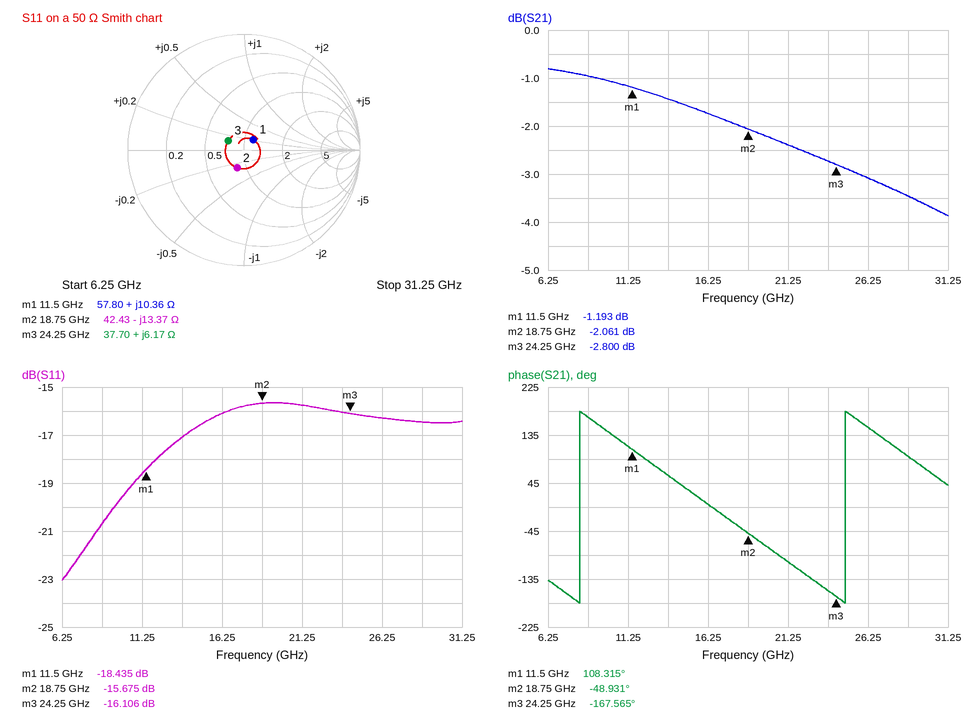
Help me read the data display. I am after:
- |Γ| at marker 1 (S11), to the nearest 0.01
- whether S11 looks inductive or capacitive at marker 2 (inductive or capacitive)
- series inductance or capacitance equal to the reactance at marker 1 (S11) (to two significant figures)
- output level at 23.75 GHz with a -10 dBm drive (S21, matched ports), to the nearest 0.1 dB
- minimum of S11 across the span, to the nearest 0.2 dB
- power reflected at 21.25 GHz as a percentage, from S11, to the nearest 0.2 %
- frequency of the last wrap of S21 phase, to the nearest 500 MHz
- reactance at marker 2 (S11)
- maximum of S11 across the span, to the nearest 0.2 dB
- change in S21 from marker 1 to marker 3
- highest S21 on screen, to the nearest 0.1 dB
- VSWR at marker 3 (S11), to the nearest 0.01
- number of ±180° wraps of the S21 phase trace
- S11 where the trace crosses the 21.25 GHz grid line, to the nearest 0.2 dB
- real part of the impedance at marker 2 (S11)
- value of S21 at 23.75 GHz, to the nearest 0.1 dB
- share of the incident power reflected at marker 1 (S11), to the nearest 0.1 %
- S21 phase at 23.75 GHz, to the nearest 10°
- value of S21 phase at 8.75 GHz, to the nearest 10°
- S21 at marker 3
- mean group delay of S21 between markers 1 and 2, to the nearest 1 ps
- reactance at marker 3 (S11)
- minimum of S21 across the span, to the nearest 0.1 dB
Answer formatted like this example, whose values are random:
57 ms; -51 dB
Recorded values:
0.12; capacitive; 140 pH; -12.7 dBm; -23.0 dB; 2.6 %; 25.0 GHz; -13.37 Ω; -15.6 dB; -1.607 dB; -0.8 dB; 1.37; 2; -15.8 dB; 42.43 Ω; -2.7 dB; 1.4 %; -160°; 170°; -2.800 dB; 60 ps; +6.17 Ω; -3.9 dB
